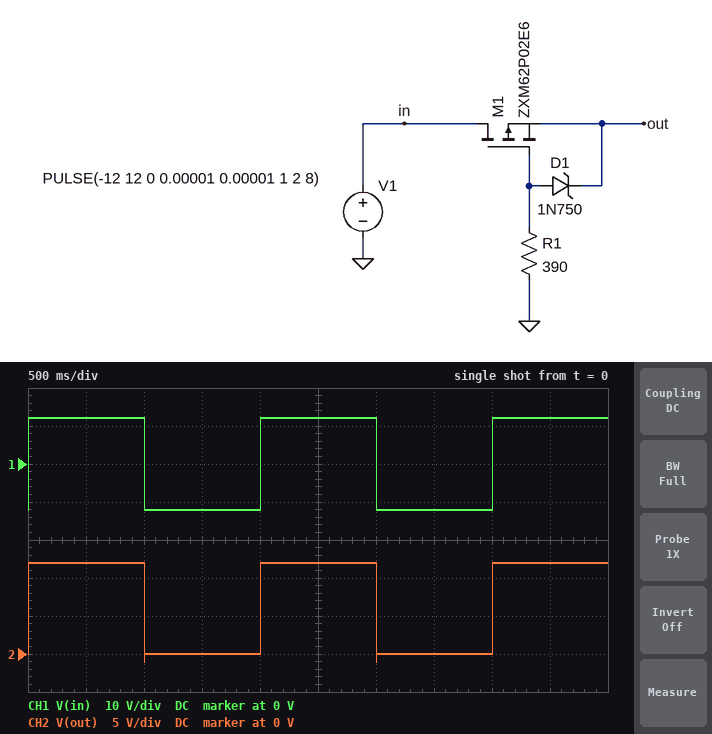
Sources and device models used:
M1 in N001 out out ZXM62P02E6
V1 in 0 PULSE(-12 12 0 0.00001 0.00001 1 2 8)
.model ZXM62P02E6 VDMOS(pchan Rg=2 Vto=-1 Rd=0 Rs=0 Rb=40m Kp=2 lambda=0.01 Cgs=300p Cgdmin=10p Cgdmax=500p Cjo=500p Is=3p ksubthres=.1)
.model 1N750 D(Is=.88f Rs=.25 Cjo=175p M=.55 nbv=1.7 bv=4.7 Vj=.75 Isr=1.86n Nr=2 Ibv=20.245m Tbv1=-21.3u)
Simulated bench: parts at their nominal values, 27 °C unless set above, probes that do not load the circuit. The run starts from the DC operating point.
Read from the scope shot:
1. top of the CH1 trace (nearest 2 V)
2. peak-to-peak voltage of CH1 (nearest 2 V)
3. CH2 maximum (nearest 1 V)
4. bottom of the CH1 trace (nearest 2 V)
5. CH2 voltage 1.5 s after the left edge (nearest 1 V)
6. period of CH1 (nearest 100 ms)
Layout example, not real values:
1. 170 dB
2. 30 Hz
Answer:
1. 12 V
2. 24 V
3. 12 V
4. -12 V
5. 0 V
6. 2.0 s
